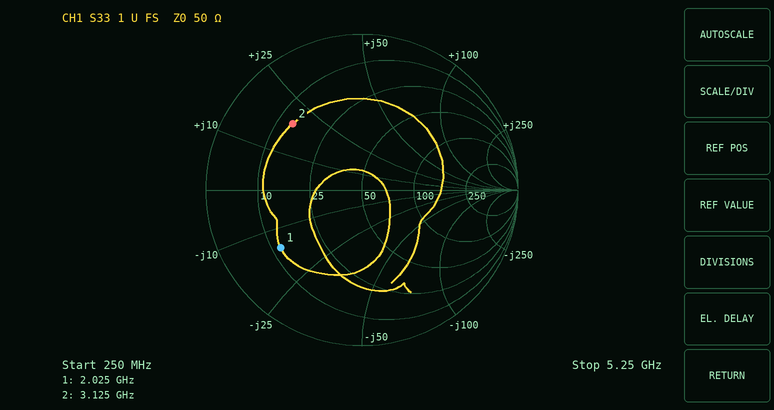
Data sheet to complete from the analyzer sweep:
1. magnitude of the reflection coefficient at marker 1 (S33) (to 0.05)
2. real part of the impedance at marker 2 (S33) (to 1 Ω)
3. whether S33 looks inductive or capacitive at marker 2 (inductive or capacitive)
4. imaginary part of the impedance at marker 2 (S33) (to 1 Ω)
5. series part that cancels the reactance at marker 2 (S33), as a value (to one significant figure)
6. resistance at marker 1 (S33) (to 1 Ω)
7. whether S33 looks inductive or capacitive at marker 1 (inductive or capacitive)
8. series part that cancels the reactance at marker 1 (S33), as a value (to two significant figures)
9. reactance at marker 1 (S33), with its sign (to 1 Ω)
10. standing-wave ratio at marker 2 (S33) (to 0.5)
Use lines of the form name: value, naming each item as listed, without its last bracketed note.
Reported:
magnitude of the reflection coefficient at marker 1 (S33): 0.65
real part of the impedance at marker 2 (S33): 14 Ω
whether S33 looks inductive or capacitive at marker 2: inductive
imaginary part of the impedance at marker 2 (S33): +19 Ω
series part that cancels the reactance at marker 2 (S33), as a value: 3 pF
resistance at marker 1 (S33): 12 Ω
whether S33 looks inductive or capacitive at marker 1: capacitive
series part that cancels the reactance at marker 1 (S33), as a value: 1.2 nH
reactance at marker 1 (S33), with its sign: -15 Ω
standing-wave ratio at marker 2 (S33): 4.0
